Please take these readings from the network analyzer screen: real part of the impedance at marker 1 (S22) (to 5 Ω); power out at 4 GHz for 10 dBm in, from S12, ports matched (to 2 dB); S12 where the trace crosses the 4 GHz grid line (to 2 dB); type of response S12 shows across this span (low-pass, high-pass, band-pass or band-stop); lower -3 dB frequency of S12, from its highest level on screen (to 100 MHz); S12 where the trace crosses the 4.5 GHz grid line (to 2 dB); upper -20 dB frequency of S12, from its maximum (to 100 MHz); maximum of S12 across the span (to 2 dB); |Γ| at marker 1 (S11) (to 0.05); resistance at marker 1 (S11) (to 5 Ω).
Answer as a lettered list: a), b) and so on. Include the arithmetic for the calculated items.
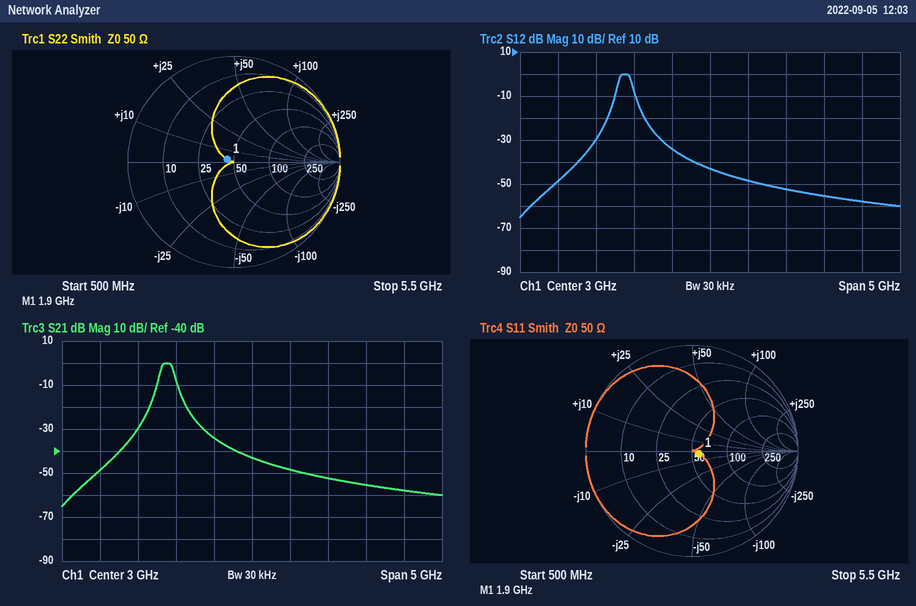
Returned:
a) 45 Ω
b) 10 dBm + (-52 dB) = -42 dBm
c) -52 dB
d) band-pass
e) 1.8 GHz
f) -56 dB
g) 2.1 GHz
h) 0 dB
i) 0.05
j) 55 Ω
